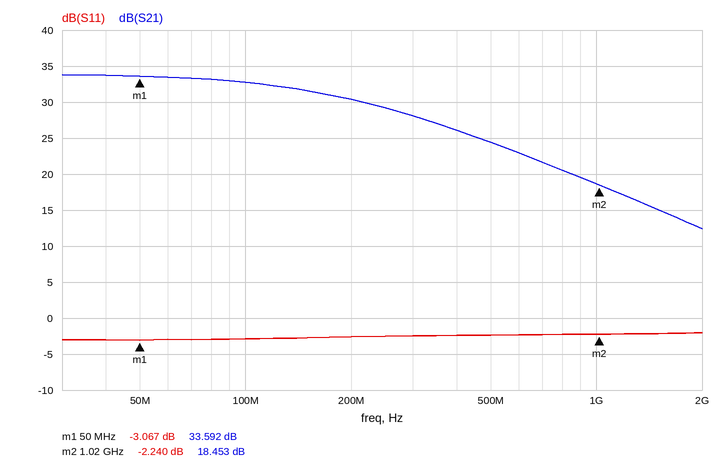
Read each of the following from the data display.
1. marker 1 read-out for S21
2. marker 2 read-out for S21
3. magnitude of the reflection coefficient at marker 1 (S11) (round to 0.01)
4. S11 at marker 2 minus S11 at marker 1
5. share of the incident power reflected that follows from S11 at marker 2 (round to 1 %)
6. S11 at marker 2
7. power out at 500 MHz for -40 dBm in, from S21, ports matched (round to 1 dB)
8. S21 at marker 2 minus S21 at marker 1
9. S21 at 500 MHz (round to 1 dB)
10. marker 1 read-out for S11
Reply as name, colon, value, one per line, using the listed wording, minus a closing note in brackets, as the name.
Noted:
marker 1 read-out for S21: 33.592 dB
marker 2 read-out for S21: 18.453 dB
magnitude of the reflection coefficient at marker 1 (S11): 0.70
S11 at marker 2 minus S11 at marker 1: 0.827 dB
share of the incident power reflected that follows from S11 at marker 2: 60 %
S11 at marker 2: -2.240 dB
power out at 500 MHz for -40 dBm in, from S21, ports matched: -16 dBm
S21 at marker 2 minus S21 at marker 1: -15.139 dB
S21 at 500 MHz: 24 dB
marker 1 read-out for S11: -3.067 dB
